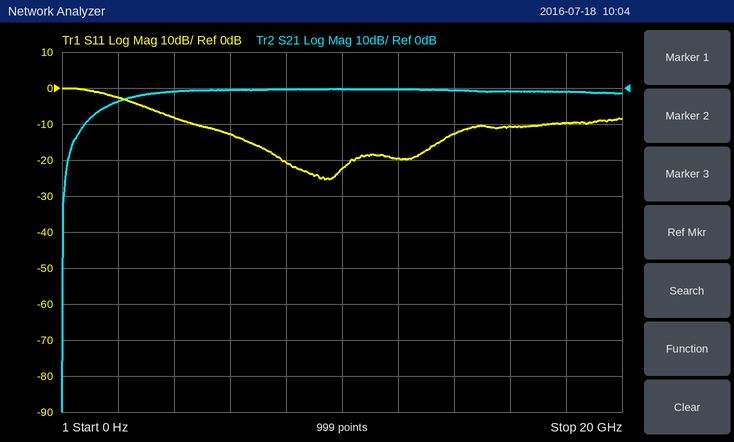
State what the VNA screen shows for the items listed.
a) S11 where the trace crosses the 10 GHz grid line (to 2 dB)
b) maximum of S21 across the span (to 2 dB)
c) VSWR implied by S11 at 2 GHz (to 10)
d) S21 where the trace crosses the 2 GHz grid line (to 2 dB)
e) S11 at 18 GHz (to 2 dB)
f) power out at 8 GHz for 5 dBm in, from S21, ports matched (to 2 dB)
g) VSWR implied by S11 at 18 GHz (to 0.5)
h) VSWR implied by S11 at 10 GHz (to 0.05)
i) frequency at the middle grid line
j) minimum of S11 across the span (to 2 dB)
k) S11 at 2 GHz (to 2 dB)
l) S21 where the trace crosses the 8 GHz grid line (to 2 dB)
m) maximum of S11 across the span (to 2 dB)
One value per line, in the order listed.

-22 dB
0 dB
10
-4 dB
-10 dB
4 dBm
2.0
1.15
10 GHz
-26 dB
-2 dB
0 dB
0 dB
